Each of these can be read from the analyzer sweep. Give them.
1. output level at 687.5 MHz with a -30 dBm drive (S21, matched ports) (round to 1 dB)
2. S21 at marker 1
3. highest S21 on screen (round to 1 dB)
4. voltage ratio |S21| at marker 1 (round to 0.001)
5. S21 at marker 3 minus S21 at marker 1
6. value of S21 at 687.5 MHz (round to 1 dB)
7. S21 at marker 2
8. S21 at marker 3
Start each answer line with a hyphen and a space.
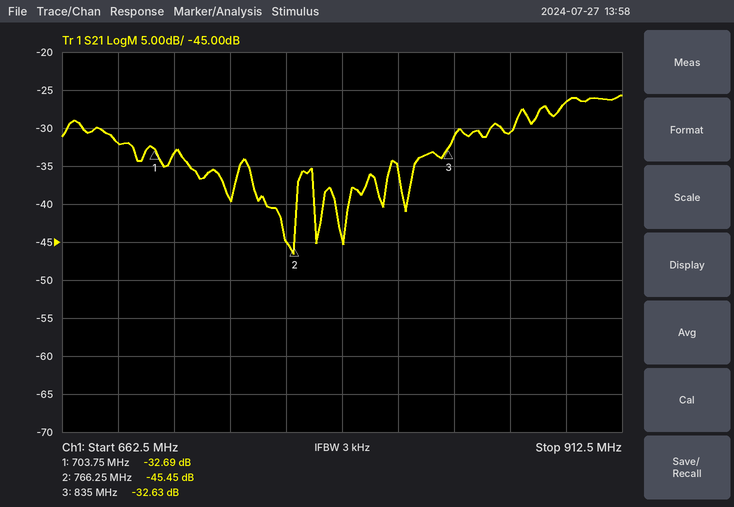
- -62 dBm
- -32.69 dB
- -26 dB
- 0.023
- 0.06 dB
- -32 dB
- -45.45 dB
- -32.63 dB
